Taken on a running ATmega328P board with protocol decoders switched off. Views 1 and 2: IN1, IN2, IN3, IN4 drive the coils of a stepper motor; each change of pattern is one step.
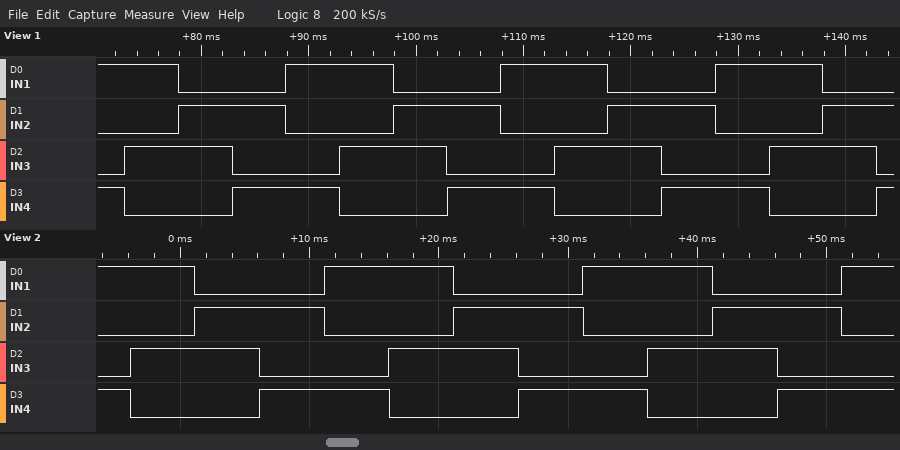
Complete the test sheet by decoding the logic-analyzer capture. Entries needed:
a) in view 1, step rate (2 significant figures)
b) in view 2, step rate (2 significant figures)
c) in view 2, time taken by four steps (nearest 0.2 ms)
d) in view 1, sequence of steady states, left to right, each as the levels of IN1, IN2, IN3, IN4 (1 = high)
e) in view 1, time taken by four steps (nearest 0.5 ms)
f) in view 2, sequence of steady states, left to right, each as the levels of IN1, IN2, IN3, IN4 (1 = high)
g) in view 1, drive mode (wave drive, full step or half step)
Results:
200 steps/s
200 steps/s
20.0 ms
1001 1010 0110 0101 1001 1010 0110 0101 1001 1010 0110 0101 1001 1010 0110 0101
20.0 ms
1001 1010 0110 0101 1001 1010 0110 0101 1001 1010 0110 0101 1001
full step
